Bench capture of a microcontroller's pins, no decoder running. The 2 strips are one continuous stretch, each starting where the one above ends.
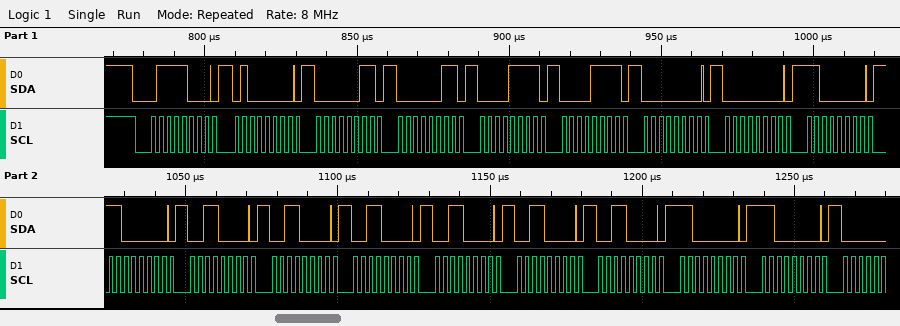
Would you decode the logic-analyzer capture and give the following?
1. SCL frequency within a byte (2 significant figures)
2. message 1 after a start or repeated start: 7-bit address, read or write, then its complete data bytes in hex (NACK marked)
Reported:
400 kHz
0x3C write: 40 03 03 0F 0F 00 00 C0 C0 30 30 30 30 30 30 C0 C0
